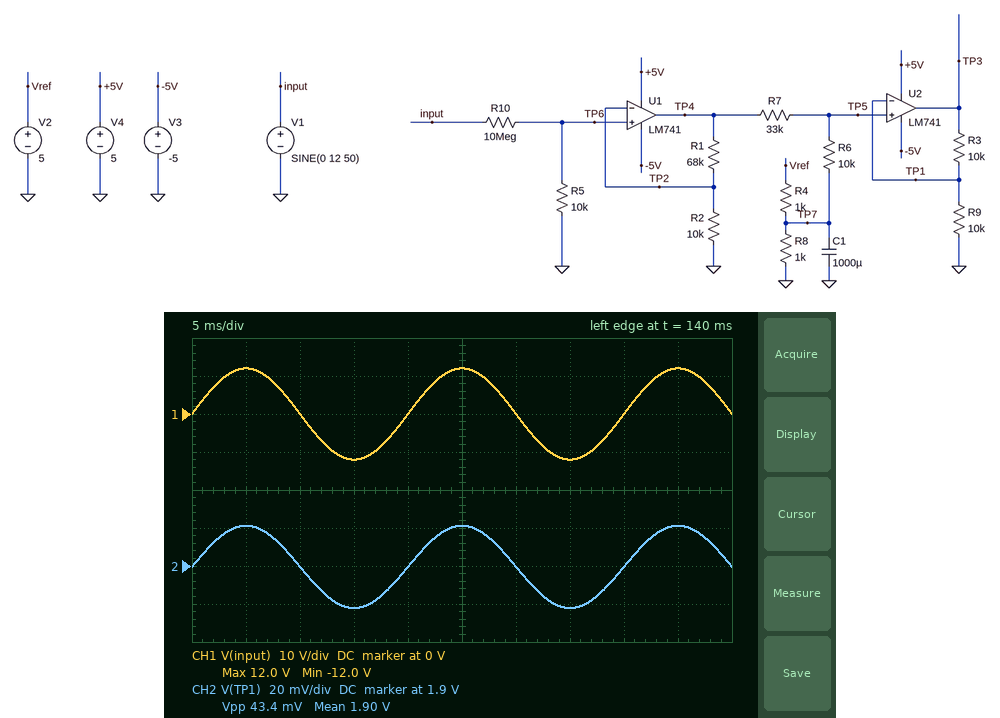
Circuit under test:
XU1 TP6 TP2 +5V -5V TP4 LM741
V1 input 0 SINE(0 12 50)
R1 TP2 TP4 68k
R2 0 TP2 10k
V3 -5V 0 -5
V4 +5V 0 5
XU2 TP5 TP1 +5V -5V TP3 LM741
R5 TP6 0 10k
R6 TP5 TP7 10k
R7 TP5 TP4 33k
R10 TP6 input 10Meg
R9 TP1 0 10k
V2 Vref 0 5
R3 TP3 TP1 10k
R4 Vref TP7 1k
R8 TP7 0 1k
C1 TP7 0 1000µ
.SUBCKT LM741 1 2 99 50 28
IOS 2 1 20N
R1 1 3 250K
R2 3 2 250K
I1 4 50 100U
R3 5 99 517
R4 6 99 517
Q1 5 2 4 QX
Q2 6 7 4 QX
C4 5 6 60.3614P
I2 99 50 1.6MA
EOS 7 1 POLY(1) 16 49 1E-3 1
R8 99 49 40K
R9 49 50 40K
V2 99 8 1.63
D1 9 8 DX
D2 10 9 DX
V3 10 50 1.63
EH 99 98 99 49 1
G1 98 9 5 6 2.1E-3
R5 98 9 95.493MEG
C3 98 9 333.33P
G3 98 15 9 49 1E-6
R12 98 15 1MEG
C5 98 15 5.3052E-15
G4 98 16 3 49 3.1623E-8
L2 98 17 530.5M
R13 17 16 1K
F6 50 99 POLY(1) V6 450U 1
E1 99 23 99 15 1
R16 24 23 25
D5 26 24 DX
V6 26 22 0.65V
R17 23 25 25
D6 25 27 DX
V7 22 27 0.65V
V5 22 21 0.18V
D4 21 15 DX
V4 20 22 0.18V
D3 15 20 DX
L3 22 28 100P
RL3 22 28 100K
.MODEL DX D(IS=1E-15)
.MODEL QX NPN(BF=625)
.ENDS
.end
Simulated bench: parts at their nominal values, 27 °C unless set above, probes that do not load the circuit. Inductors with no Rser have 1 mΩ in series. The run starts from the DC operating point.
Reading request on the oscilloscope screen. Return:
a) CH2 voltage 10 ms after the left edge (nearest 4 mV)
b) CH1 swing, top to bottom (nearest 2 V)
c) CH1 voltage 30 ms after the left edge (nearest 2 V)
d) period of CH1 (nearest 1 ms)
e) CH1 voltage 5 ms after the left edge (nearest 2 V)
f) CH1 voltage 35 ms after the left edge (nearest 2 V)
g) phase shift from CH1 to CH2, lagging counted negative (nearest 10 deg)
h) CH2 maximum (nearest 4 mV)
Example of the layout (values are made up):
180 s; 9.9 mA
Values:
1.900 V; 24 V; 0 V; 20 ms; 12 V; -12 V; 0 deg; 1.920 V
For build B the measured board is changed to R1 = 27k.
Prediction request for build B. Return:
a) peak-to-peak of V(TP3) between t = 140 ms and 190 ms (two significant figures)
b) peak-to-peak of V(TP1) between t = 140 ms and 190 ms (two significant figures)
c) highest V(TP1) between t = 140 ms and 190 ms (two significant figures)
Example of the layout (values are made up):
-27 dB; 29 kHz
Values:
41 mV; 21 mV; 1.9 V
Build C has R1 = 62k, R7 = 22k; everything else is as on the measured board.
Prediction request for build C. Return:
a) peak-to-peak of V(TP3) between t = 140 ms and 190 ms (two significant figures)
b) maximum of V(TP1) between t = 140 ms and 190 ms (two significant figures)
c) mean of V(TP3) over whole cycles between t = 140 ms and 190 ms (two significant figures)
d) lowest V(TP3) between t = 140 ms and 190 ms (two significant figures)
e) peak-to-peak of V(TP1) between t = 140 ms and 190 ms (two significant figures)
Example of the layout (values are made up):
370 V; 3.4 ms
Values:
110 mV; 1.7 V; 3.4 V; 3.3 V; 54 mV
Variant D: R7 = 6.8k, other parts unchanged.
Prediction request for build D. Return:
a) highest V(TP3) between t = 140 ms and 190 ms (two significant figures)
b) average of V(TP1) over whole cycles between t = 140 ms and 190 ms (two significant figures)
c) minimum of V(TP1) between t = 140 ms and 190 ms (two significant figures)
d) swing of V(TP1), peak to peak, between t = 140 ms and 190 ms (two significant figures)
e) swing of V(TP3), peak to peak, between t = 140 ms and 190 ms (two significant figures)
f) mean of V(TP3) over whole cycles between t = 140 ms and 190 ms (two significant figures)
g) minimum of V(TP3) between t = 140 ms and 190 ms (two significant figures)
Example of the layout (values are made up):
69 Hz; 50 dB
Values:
2.1 V; 990 mV; 930 mV; 110 mV; 220 mV; 2.0 V; 1.9 V
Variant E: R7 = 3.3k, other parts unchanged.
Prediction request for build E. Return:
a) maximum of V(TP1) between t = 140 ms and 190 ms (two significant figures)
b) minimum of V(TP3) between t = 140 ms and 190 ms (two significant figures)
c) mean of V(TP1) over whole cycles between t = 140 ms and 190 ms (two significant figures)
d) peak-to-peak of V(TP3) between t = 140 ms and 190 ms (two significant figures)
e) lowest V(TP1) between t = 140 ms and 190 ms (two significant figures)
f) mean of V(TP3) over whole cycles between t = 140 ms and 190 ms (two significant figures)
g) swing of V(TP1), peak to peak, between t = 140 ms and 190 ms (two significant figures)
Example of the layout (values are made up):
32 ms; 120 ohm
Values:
680 mV; 1.1 V; 610 mV; 280 mV; 540 mV; 1.2 V; 140 mV
